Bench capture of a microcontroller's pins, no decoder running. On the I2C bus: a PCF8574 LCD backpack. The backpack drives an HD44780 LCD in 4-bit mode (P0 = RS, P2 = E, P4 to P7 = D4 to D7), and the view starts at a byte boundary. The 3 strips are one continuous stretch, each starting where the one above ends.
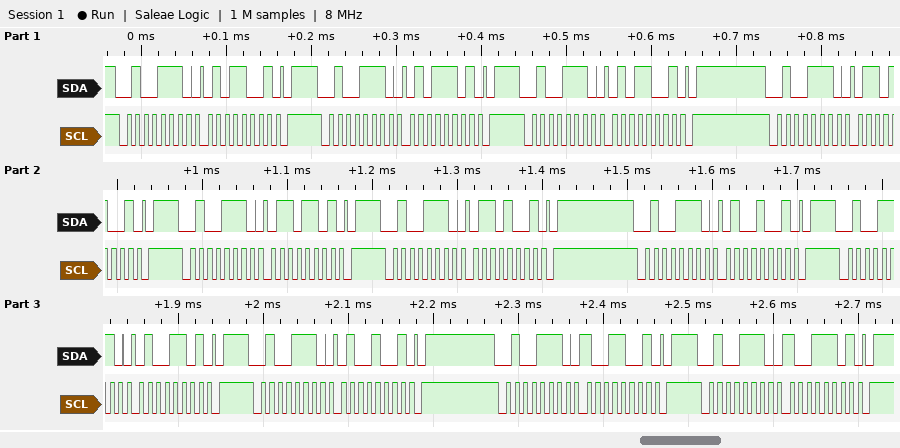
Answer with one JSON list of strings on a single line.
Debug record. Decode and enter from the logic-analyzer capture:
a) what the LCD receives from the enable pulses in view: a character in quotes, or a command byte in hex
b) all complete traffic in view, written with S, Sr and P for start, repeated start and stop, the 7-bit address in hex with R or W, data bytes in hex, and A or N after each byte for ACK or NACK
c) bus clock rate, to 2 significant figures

["'V'", "S 27W A 59 A P S 27W A 5D A P S 27W A 59 A P S 27W A 69 A P S 27W A 6D A P S 27W A 69 A P S 27W A 49 A P S 27W A 4D A P S 27W A 49 A P S 27W A 99 A P S 27W A 9D A P", "100 kHz"]
